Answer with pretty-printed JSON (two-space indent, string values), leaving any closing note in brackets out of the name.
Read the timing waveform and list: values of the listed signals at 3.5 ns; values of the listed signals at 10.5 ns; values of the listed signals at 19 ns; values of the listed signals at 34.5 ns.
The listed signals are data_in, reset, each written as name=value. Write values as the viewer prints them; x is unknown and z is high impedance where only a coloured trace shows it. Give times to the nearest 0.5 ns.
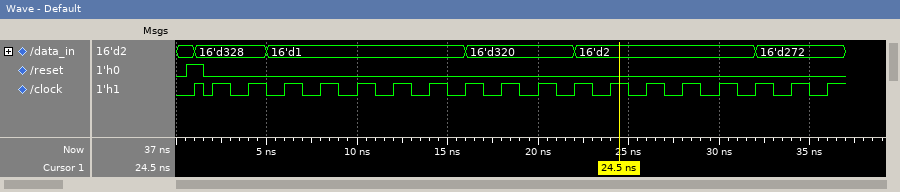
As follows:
{
  "values of the listed signals at 3.5 ns": "data_in=16'd328, reset=0",
  "values of the listed signals at 10.5 ns": "data_in=16'd1, reset=0",
  "values of the listed signals at 19 ns": "data_in=16'd320, reset=0",
  "values of the listed signals at 34.5 ns": "data_in=16'd272, reset=0"
}
